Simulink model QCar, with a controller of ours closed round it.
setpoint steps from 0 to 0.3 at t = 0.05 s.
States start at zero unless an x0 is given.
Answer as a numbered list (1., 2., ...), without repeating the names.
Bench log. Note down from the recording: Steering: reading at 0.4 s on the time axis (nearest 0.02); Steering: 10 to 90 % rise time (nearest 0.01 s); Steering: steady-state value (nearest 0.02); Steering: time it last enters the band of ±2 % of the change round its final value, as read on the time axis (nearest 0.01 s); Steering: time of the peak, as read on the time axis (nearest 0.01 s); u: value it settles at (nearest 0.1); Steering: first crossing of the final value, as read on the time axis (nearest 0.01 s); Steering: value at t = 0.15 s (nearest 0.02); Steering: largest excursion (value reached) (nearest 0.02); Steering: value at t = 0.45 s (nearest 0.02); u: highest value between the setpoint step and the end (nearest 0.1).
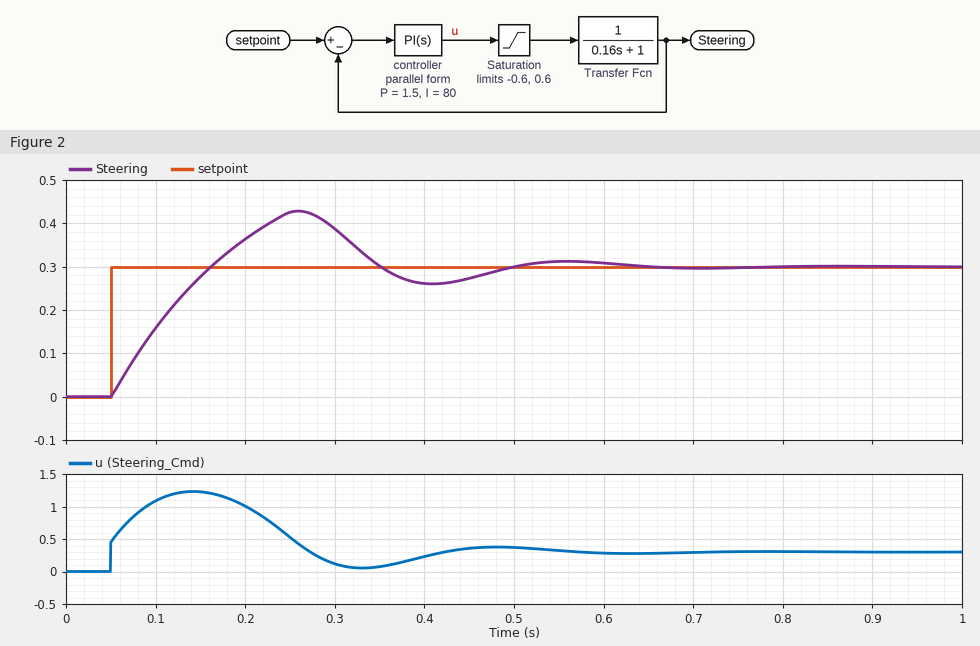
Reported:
1. 0.26
2. 0.09 s
3. 0.30
4. 0.61 s
5. 0.26 s
6. 0.3
7. 0.16 s
8. 0.28
9. 0.42
10. 0.28
11. 1.2
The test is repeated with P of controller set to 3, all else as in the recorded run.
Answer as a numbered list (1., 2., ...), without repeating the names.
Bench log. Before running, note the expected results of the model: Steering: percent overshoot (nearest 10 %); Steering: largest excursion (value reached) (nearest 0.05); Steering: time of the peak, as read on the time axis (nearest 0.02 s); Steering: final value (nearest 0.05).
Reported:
1. 40 %
2. 0.40
3. 0.24 s
4. 0.30
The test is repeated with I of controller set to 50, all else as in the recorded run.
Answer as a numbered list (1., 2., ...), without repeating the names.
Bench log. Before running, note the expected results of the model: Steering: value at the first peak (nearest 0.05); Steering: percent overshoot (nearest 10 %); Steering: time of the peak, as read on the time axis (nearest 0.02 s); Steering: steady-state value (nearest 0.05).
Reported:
1. 0.40
2. 30 %
3. 0.24 s
4. 0.30
